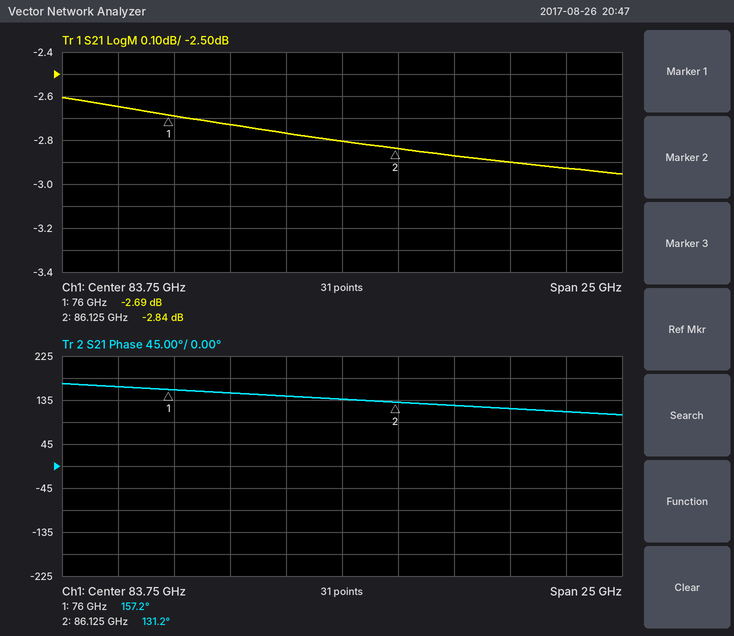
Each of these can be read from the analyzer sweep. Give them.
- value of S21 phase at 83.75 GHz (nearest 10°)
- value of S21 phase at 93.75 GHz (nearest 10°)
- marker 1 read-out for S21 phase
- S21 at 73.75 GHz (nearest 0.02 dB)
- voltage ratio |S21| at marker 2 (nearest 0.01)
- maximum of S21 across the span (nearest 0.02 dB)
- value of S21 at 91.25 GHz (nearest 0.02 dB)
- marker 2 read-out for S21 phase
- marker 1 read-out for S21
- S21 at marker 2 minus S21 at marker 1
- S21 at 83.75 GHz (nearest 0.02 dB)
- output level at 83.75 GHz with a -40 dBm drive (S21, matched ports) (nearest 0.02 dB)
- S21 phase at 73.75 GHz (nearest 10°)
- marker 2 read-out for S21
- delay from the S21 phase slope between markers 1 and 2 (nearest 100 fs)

140°
110°
157.2°
-2.64 dB
0.72
-2.60 dB
-2.90 dB
131.2°
-2.69 dB
-0.15 dB
-2.80 dB
-42.80 dBm
160°
-2.84 dB
7.1 ps
